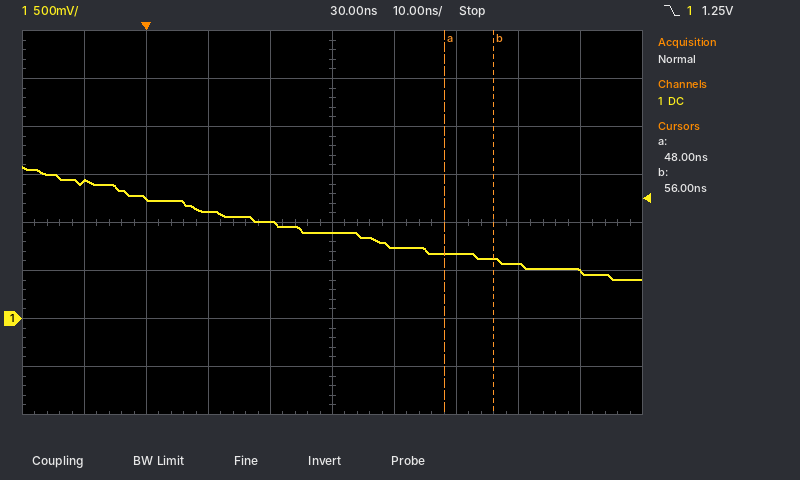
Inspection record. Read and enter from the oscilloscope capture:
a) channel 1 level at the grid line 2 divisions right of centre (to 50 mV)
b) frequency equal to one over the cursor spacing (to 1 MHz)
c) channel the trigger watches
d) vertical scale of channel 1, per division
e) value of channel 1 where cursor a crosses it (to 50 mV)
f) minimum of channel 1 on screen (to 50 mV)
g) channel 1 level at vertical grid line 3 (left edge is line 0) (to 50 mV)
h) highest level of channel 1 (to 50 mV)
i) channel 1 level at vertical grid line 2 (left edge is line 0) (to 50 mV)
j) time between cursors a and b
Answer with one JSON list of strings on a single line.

["700 mV", "125 MHz", "channel 1", "500 mV", "700 mV", "400 mV", "1.10 V", "1.60 V", "1.25 V", "8 ns"]
